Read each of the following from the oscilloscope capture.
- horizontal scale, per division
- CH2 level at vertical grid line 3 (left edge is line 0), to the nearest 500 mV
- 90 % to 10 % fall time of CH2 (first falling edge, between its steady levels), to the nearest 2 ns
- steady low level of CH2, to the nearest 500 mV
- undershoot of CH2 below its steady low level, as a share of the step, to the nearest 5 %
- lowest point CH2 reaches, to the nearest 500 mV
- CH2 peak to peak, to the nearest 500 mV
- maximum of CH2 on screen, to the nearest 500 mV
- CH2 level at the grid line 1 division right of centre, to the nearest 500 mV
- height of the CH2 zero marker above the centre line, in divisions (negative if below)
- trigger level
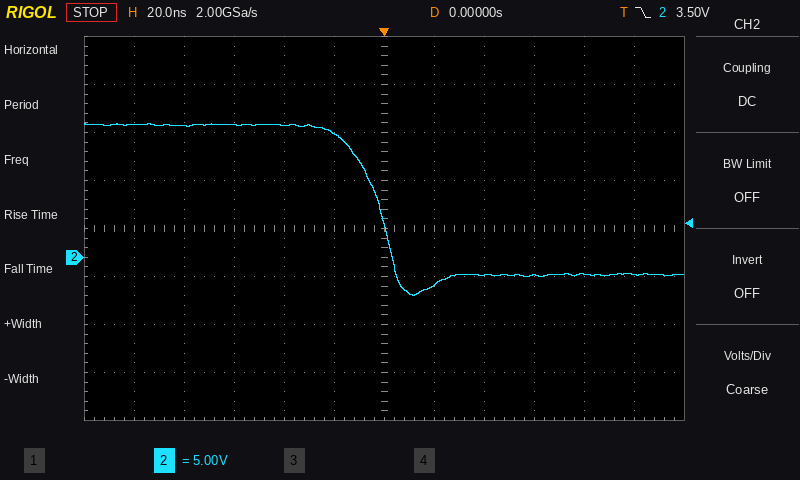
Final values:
20 ns
14.0 V
20 ns
-2.0 V
15 %
-4.0 V
18.0 V
14.0 V
-3.0 V
-0.6 div
3.50 V
